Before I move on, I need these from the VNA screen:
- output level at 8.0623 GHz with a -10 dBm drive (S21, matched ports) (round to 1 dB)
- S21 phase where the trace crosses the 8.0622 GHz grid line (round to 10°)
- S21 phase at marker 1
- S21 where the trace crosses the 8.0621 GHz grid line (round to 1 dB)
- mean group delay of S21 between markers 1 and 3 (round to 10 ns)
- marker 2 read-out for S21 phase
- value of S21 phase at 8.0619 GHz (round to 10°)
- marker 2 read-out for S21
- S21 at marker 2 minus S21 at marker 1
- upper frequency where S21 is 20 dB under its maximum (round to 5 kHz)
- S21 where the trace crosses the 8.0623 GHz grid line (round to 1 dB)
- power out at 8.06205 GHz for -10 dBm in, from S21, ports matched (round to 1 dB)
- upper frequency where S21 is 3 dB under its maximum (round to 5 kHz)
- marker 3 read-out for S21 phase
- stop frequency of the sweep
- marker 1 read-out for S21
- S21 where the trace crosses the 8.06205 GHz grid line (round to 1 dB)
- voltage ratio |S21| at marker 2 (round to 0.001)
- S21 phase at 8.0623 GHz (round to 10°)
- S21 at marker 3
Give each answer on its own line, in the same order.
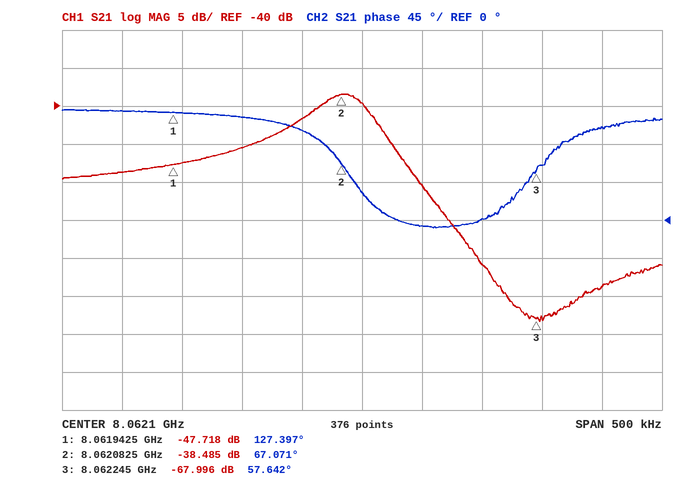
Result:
-74 dBm
0°
127.397°
-40 dB
640 ns
67.071°
130°
-38.485 dB
9.233 dB
8.062190 GHz
-64 dB
-52 dBm
8.062110 GHz
57.642°
8.06235 GHz
-47.718 dB
-42 dB
0.012
110°
-67.996 dB
